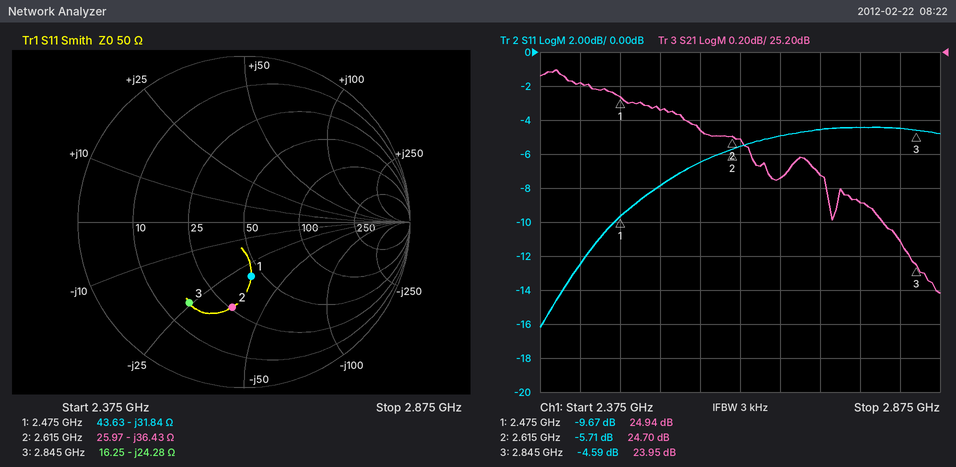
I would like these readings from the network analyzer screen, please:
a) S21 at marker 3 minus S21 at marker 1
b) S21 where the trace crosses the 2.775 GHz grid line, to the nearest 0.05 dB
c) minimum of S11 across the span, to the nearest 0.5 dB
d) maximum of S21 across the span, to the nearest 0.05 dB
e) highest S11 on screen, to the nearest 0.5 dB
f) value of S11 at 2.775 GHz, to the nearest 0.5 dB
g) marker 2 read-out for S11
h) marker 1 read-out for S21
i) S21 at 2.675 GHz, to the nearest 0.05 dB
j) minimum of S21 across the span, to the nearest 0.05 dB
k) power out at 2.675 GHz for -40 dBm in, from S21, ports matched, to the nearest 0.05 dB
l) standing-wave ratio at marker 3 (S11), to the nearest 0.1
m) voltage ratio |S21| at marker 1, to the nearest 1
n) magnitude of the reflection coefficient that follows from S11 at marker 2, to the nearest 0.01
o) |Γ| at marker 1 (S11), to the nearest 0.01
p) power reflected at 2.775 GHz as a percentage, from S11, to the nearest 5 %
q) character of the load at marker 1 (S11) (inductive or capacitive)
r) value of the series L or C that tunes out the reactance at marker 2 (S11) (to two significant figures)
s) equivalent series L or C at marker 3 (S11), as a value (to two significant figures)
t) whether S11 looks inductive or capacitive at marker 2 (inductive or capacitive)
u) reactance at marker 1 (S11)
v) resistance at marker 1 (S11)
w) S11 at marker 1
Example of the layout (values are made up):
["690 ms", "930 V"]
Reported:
["-0.99 dB", "24.30 dB", "-16.0 dB", "25.10 dB", "-4.5 dB", "-4.5 dB", "-5.71 dB", "24.94 dB", "24.45 dB", "23.80 dB", "-15.55 dBm", "3.9", "18", "0.52", "0.33", "35 %", "capacitive", "2.2 nH", "2.3 pF", "capacitive", "-31.84 Ω", "43.63 Ω", "-9.67 dB"]
